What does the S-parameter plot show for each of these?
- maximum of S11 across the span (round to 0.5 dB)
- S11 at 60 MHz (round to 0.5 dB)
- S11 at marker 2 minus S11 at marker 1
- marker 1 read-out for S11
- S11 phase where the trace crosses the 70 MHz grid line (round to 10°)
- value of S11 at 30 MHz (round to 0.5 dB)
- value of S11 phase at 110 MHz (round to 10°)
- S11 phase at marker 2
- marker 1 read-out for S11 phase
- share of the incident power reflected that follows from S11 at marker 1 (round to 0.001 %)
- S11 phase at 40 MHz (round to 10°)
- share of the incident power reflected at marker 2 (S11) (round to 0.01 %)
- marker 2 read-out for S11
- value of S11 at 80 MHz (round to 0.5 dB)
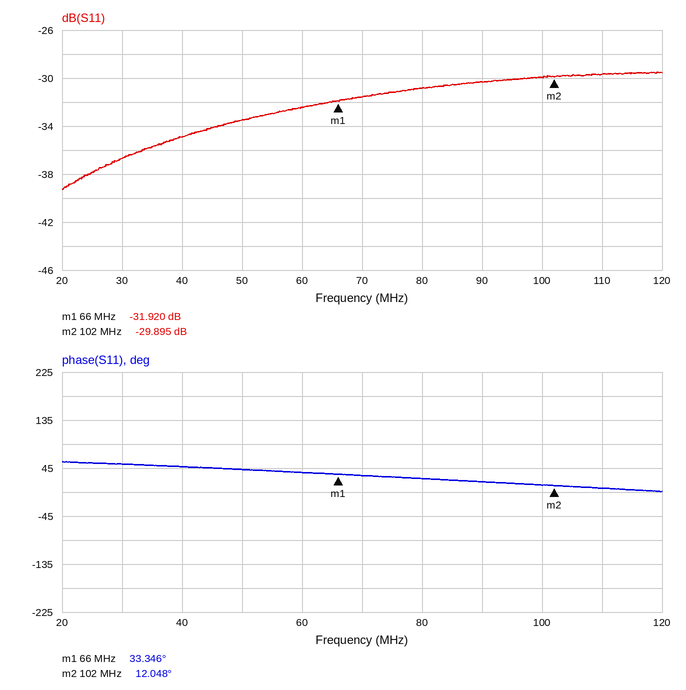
-29.5 dB
-32.5 dB
2.025 dB
-31.920 dB
30°
-36.5 dB
10°
12.048°
33.346°
0.064 %
50°
0.10 %
-29.895 dB
-31.0 dB
